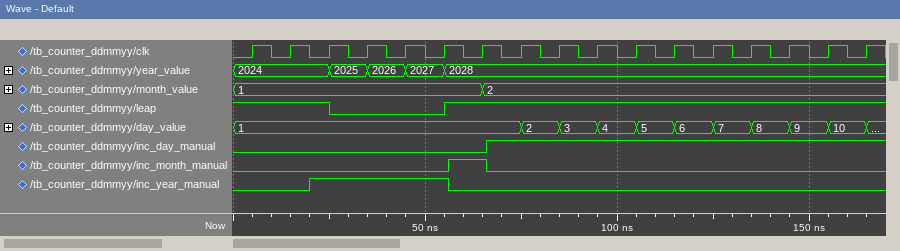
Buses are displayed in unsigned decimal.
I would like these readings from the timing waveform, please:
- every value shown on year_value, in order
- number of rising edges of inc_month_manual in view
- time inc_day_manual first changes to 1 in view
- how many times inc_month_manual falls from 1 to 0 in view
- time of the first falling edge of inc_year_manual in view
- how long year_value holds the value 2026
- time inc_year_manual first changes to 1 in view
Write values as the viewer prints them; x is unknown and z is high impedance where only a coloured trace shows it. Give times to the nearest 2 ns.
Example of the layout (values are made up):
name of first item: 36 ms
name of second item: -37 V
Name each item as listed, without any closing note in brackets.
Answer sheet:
every value shown on year_value, in order: 2024, 2025, 2026, 2027, 2028
number of rising edges of inc_month_manual in view: 1
time inc_day_manual first changes to 1 in view: 66 ns
how many times inc_month_manual falls from 1 to 0 in view: 1
time of the first falling edge of inc_year_manual in view: 56 ns
how long year_value holds the value 2026: 10 ns
time inc_year_manual first changes to 1 in view: 20 ns
